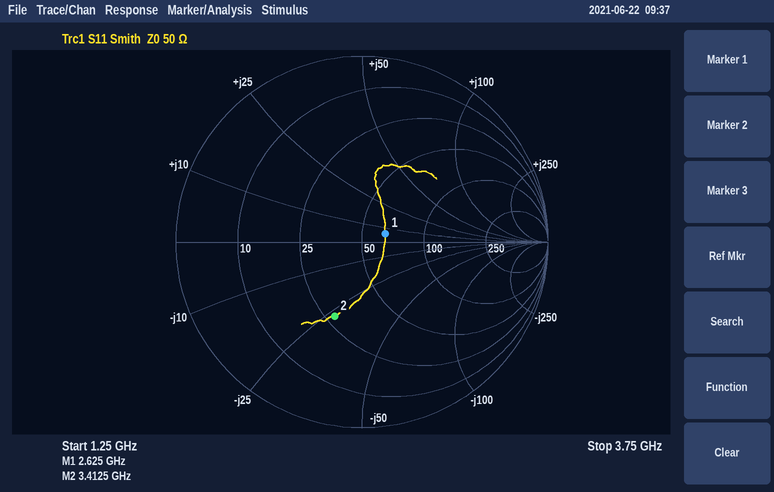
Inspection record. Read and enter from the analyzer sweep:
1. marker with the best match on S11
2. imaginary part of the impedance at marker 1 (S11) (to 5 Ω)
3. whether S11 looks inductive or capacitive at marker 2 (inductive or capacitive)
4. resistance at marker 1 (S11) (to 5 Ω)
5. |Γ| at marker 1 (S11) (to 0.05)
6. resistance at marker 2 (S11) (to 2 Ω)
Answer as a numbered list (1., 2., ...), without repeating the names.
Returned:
1. marker 1
2. +5 Ω
3. capacitive
4. 65 Ω
5. 0.15
6. 28 Ω
